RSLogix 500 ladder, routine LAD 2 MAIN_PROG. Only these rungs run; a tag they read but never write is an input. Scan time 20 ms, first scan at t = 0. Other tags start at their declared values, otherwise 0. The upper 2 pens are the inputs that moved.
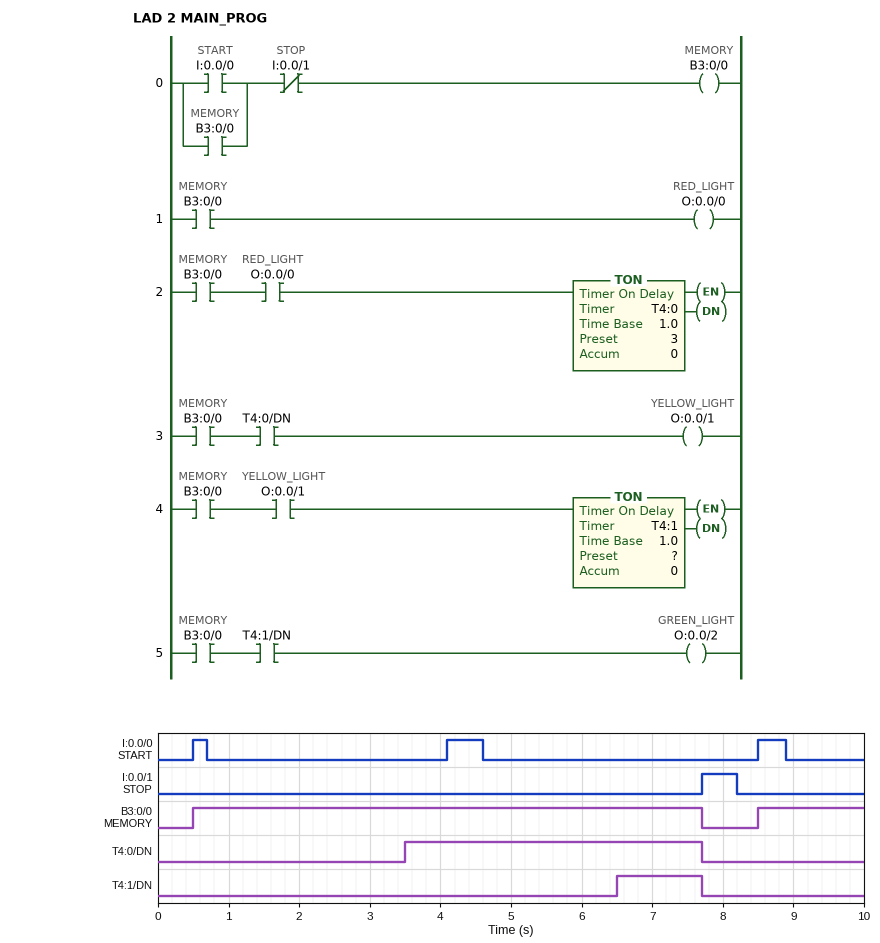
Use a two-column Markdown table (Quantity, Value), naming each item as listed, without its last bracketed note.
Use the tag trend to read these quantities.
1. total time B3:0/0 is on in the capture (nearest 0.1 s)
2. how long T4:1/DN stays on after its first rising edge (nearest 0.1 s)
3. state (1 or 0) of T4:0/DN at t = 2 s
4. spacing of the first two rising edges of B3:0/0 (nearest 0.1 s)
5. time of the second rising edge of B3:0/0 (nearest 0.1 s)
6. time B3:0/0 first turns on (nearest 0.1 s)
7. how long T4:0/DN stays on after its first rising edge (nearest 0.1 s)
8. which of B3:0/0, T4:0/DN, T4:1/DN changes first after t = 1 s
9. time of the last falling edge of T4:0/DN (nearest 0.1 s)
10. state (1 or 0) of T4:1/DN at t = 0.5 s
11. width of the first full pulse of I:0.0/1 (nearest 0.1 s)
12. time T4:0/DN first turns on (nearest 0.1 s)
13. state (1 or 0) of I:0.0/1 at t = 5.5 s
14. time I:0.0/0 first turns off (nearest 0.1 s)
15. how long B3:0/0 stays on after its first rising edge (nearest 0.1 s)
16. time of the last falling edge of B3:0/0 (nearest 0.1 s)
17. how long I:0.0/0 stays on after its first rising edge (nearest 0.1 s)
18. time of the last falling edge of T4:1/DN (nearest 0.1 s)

| Quantity | Value |
|---|---|
| total time B3:0/0 is on in the capture | 8.7 s |
| how long T4:1/DN stays on after its first rising edge | 1.2 s |
| state (1 or 0) of T4:0/DN at t = 2 s | 0 |
| spacing of the first two rising edges of B3:0/0 | 8.0 s |
| time of the second rising edge of B3:0/0 | 8.5 s |
| time B3:0/0 first turns on | 0.5 s |
| how long T4:0/DN stays on after its first rising edge | 4.2 s |
| which of B3:0/0, T4:0/DN, T4:1/DN changes first after t = 1 s | T4:0/DN |
| time of the last falling edge of T4:0/DN | 7.7 s |
| state (1 or 0) of T4:1/DN at t = 0.5 s | 0 |
| width of the first full pulse of I:0.0/1 | 0.5 s |
| time T4:0/DN first turns on | 3.5 s |
| state (1 or 0) of I:0.0/1 at t = 5.5 s | 0 |
| time I:0.0/0 first turns off | 0.7 s |
| how long B3:0/0 stays on after its first rising edge | 7.2 s |
| time of the last falling edge of B3:0/0 | 7.7 s |
| how long I:0.0/0 stays on after its first rising edge | 0.2 s |
| time of the last falling edge of T4:1/DN | 7.7 s |
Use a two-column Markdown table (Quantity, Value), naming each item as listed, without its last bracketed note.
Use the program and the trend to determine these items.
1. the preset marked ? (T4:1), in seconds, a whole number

| Quantity | Value |
|---|---|
| the preset marked ? (T4:1), in seconds, a whole number | 3 s |
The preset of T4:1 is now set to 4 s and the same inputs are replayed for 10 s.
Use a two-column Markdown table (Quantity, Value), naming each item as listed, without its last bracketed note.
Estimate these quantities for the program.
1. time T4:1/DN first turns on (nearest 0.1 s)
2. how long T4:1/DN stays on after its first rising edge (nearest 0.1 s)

| Quantity | Value |
|---|---|
| time T4:1/DN first turns on | 7.5 s |
| how long T4:1/DN stays on after its first rising edge | 0.2 s |
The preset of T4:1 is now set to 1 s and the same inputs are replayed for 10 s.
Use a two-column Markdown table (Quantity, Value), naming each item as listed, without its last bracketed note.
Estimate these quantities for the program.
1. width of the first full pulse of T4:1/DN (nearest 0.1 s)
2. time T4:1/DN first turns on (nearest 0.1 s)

| Quantity | Value |
|---|---|
| width of the first full pulse of T4:1/DN | 3.2 s |
| time T4:1/DN first turns on | 4.5 s |
